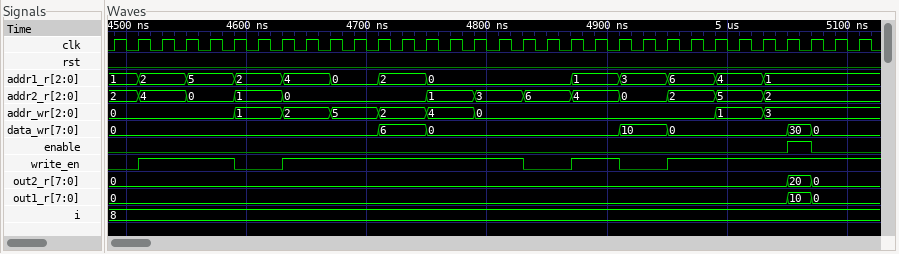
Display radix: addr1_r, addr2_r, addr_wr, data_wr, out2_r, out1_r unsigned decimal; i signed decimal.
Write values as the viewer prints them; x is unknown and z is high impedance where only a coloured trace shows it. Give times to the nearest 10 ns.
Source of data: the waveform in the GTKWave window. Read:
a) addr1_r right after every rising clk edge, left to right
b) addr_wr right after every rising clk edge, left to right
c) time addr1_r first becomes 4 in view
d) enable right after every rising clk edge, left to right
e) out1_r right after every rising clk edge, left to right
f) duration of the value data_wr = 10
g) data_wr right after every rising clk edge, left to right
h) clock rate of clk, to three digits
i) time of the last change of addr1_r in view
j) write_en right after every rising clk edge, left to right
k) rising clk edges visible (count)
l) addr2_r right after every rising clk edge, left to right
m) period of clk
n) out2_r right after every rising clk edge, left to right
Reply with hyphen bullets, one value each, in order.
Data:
- 1, 2, 2, 5, 5, 2, 2, 4, 4, 0, 0, 2, 2, 0, 0, 0, 0, 0, 0, 1, 1, 3, 3, 6, 6, 4, 4, 1, 1, 1, 1, 1
- 0, 0, 0, 0, 0, 1, 1, 2, 2, 5, 5, 2, 2, 4, 4, 0, 0, 0, 0, 0, 0, 0, 0, 0, 0, 1, 1, 3, 3, 3, 3, 3
- 4630 ns
- 0 0 0 0 0 0 0 0 0 0 0 0 0 0 0 0 0 0 0 0 0 0 0 0 0 0 0 0 1 0 0 0
- 0, 0, 0, 0, 0, 0, 0, 0, 0, 0, 0, 0, 0, 0, 0, 0, 0, 0, 0, 0, 0, 0, 0, 0, 0, 0, 0, 0, 10, 0, 0, 0
- 40 ns
- 0, 0, 0, 0, 0, 0, 0, 0, 0, 0, 0, 6, 6, 0, 0, 0, 0, 0, 0, 0, 0, 10, 10, 0, 0, 0, 0, 0, 30, 0, 0, 0
- 50.0 MHz
- 5030 ns
- 0 1 1 1 1 0 0 1 1 1 1 1 1 1 1 1 1 0 0 1 1 0 0 1 1 1 1 1 1 1 1 1
- 32
- 2, 4, 4, 0, 0, 1, 1, 0, 0, 0, 0, 0, 0, 1, 1, 3, 3, 6, 6, 4, 4, 0, 0, 2, 2, 5, 5, 2, 2, 2, 2, 2
- 20 ns
- 0, 0, 0, 0, 0, 0, 0, 0, 0, 0, 0, 0, 0, 0, 0, 0, 0, 0, 0, 0, 0, 0, 0, 0, 0, 0, 0, 0, 20, 0, 0, 0
